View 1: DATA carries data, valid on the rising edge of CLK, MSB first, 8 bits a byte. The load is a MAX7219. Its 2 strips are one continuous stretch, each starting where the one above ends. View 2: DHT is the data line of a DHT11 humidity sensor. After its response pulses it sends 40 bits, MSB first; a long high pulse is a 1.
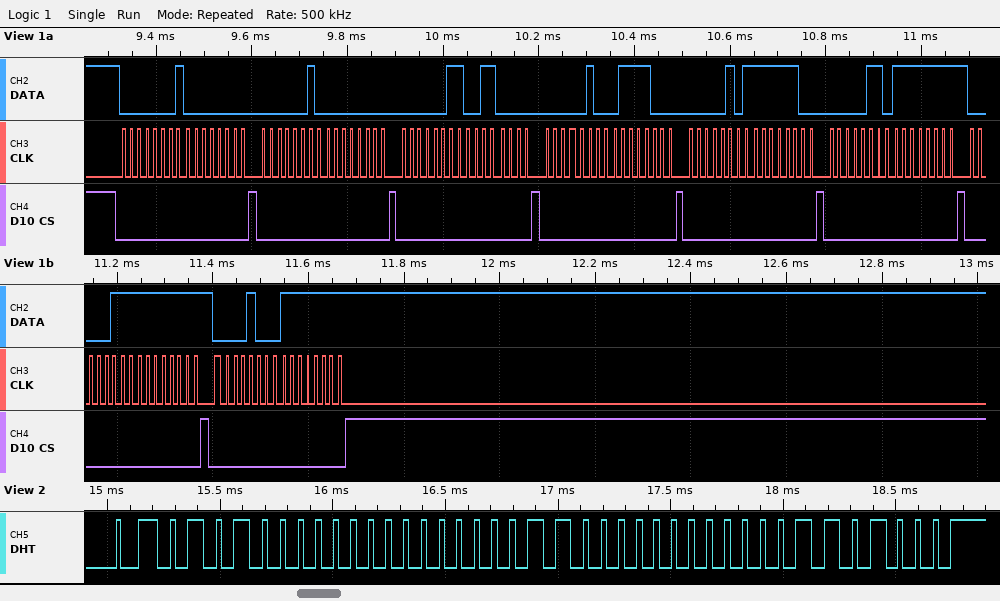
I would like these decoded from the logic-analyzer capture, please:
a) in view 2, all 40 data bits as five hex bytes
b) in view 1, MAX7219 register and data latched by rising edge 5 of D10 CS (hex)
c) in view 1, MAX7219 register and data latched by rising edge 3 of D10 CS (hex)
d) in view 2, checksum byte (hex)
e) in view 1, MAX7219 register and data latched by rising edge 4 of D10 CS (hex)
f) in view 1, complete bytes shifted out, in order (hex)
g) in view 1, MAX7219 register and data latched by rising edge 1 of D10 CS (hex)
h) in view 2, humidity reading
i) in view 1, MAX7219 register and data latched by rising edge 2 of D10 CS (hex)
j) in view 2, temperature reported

50 00 18 00 68
register 0x5, data 0xFC
register 0x3, data 0x30
0x68
register 0x4, data 0x78
01 00 02 00 03 30 04 78 05 FC 06 FF 07 FF 08 FF
register 0x1, data 0x00
80 %
register 0x2, data 0x00
24.0 °C
